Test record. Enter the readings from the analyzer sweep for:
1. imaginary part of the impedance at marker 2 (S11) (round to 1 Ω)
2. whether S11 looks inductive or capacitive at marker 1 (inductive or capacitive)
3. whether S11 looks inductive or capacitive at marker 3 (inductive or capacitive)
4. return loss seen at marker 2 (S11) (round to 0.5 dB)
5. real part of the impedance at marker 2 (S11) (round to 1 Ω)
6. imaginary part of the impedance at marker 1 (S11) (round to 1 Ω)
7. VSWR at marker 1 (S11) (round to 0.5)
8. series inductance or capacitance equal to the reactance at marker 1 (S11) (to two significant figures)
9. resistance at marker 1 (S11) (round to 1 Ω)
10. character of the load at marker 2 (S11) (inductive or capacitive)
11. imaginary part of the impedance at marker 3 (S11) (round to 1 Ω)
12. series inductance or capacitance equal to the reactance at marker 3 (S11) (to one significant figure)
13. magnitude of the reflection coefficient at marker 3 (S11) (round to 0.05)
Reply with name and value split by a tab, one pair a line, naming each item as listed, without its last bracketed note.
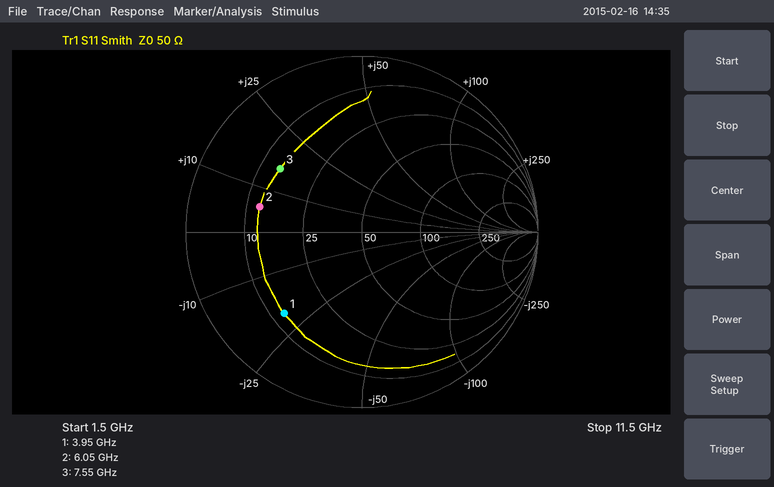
imaginary part of the impedance at marker 2 (S11)	+6 Ω
whether S11 looks inductive or capacitive at marker 1	capacitive
whether S11 looks inductive or capacitive at marker 3	inductive
return loss seen at marker 2 (S11)	4.5 dB
real part of the impedance at marker 2 (S11)	13 Ω
imaginary part of the impedance at marker 1 (S11)	-20 Ω
VSWR at marker 1 (S11)	4.5
series inductance or capacitance equal to the reactance at marker 1 (S11)	2.0 pF
resistance at marker 1 (S11)	13 Ω
character of the load at marker 2 (S11)	inductive
imaginary part of the impedance at marker 3 (S11)	+16 Ω
series inductance or capacitance equal to the reactance at marker 3 (S11)	300 pH
magnitude of the reflection coefficient at marker 3 (S11)	0.60
